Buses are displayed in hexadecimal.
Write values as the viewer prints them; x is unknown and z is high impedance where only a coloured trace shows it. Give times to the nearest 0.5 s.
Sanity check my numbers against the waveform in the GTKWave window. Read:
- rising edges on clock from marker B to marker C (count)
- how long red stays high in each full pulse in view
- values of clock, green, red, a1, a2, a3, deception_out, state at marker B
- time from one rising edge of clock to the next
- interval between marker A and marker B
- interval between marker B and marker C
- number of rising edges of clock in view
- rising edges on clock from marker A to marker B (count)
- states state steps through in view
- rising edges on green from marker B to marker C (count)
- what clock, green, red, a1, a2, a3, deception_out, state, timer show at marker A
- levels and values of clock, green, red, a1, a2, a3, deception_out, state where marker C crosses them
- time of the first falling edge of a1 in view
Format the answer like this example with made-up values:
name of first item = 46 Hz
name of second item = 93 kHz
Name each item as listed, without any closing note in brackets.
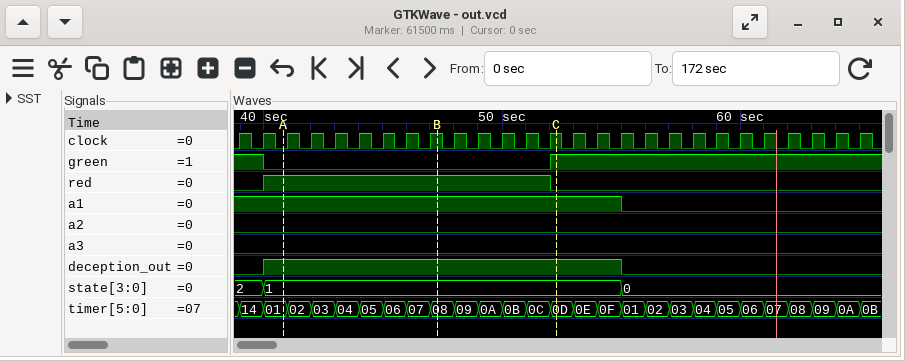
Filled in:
rising edges on clock from marker B to marker C = 5
how long red stays high in each full pulse in view = 12 s
values of clock, green, red, a1, a2, a3, deception_out, state at marker B = clock=1, green=0, red=1, a1=1, a2=0, a3=0, deception_out=1, state=1
time from one rising edge of clock to the next = 1 s
interval between marker A and marker B = 6.5 s
interval between marker B and marker C = 5 s
number of rising edges of clock in view = 27
rising edges on clock from marker A to marker B = 7
states state steps through in view = 2, 1, 0
rising edges on green from marker B to marker C = 1
what clock, green, red, a1, a2, a3, deception_out, state, timer show at marker A = clock=0, green=0, red=1, a1=1, a2=0, a3=0, deception_out=1, state=1, timer=01
levels and values of clock, green, red, a1, a2, a3, deception_out, state where marker C crosses them = clock=1, green=1, red=0, a1=1, a2=0, a3=0, deception_out=1, state=1
time of the first falling edge of a1 in view = 55 s
